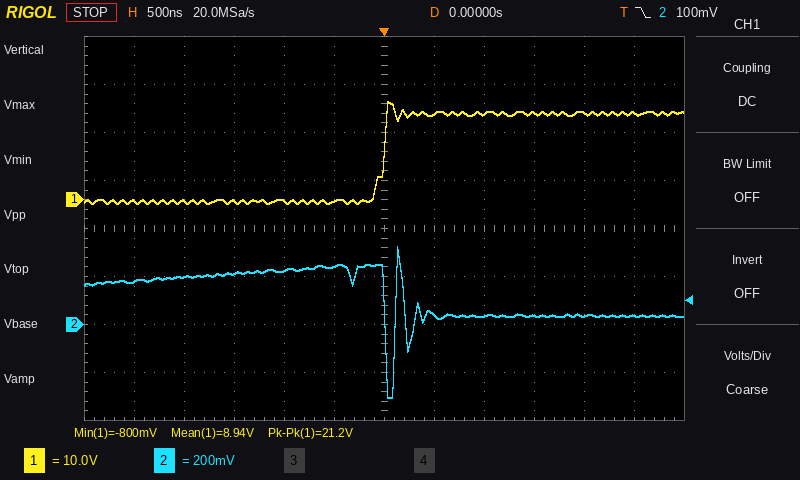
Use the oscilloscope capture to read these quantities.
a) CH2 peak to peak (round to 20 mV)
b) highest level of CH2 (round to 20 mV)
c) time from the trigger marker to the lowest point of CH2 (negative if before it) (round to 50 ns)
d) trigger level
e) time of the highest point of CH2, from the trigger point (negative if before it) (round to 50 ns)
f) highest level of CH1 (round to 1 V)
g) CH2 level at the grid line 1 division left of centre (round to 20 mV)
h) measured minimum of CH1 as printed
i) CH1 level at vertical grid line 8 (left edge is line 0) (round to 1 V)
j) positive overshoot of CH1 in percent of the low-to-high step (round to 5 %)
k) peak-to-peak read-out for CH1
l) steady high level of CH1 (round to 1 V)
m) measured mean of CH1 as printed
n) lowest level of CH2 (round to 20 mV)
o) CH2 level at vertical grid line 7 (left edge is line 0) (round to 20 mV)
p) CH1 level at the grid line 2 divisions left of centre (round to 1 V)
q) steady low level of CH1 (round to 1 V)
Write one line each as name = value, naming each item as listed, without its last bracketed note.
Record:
CH2 peak to peak = 620 mV
highest level of CH2 = 320 mV
time from the trigger marker to the lowest point of CH2 (negative if before it) = +50 ns
trigger level = 100 mV
time of the highest point of CH2, from the trigger point (negative if before it) = +150 ns
highest level of CH1 = 20 V
CH2 level at the grid line 1 division left of centre = 240 mV
measured minimum of CH1 as printed = -800 mV
CH1 level at vertical grid line 8 (left edge is line 0) = 18 V
positive overshoot of CH1 in percent of the low-to-high step = 10 %
peak-to-peak read-out for CH1 = 21.2 V
steady high level of CH1 = 18 V
measured mean of CH1 as printed = 8.94 V
lowest level of CH2 = -300 mV
CH2 level at vertical grid line 7 (left edge is line 0) = 40 mV
CH1 level at the grid line 2 divisions left of centre = 0 V
steady low level of CH1 = 0 V
